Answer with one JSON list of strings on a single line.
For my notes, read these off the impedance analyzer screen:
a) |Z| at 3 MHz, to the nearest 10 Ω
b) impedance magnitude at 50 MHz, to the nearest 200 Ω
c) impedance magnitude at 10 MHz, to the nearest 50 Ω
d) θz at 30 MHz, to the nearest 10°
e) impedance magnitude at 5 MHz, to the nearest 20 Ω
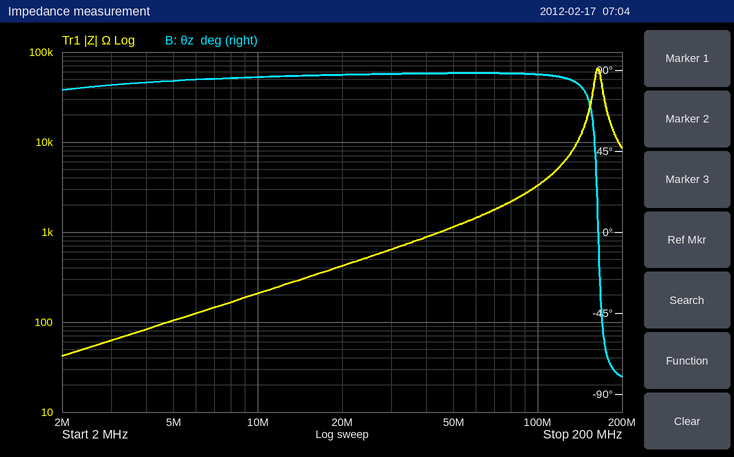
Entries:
["60 Ω", "1.2 kΩ", "200 Ω", "90°", "100 Ω"]
